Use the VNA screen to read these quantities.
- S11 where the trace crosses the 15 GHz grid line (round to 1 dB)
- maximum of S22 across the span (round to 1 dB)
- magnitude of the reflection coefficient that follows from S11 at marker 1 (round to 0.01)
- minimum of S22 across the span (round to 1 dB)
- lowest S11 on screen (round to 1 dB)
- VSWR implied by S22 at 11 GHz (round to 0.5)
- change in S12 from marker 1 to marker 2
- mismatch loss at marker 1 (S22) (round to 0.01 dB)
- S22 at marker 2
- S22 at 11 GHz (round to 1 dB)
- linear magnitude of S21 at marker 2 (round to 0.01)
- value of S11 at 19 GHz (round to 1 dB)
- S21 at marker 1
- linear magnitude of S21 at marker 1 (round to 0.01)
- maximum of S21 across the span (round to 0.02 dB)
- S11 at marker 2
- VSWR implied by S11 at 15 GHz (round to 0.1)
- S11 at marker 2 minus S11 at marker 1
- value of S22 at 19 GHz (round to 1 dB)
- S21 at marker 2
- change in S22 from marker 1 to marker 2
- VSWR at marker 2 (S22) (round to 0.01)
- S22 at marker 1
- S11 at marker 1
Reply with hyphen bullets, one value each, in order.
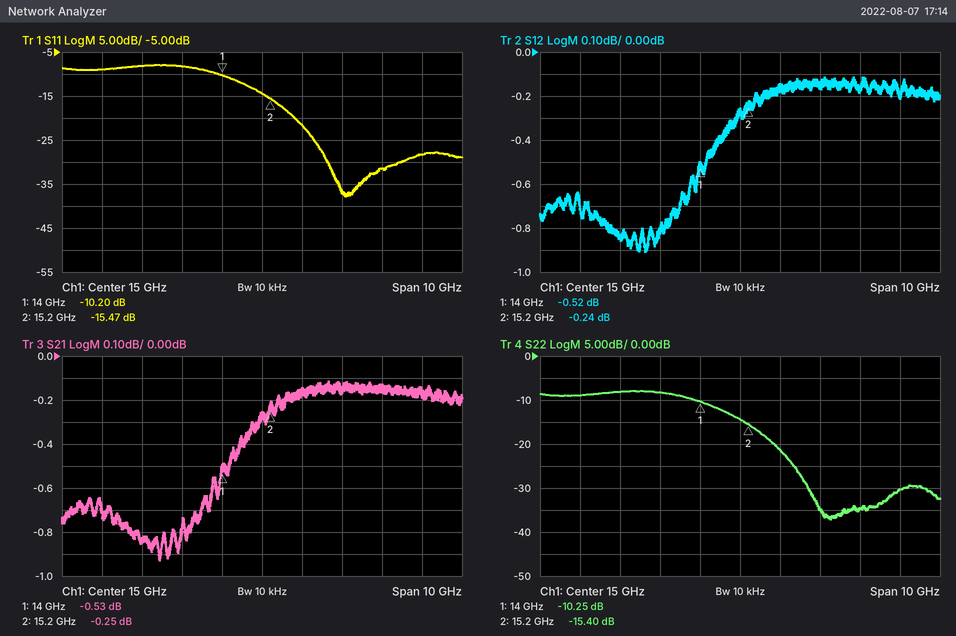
- -14 dB
- -8 dB
- 0.31
- -37 dB
- -38 dB
- 2.0
- 0.28 dB
- 0.43 dB
- -15.40 dB
- -9 dB
- 0.97
- -28 dB
- -0.53 dB
- 0.94
- -0.12 dB
- -15.47 dB
- 1.5
- -5.27 dB
- -30 dB
- -0.25 dB
- -5.15 dB
- 1.41
- -10.25 dB
- -10.20 dB
